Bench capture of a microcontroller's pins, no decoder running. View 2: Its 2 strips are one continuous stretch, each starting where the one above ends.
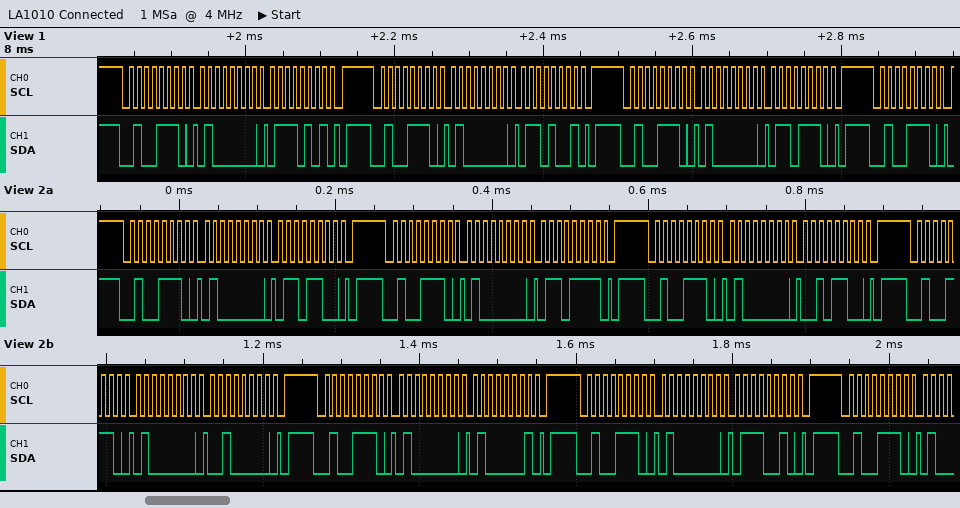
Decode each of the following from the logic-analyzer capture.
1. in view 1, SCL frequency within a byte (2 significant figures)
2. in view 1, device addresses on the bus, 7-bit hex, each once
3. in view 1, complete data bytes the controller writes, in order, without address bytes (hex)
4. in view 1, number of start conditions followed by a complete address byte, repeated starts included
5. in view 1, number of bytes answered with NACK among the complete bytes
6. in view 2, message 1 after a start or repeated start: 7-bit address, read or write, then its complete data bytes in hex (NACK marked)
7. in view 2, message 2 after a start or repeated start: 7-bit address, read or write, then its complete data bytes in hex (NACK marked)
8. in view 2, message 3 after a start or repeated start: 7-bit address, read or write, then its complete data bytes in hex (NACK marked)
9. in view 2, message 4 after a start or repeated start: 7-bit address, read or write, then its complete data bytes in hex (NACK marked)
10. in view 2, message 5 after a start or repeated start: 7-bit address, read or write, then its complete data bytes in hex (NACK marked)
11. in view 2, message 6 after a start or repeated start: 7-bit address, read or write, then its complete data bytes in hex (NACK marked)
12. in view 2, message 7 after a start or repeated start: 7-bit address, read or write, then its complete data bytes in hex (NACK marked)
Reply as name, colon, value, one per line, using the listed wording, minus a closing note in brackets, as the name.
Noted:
in view 1, SCL frequency within a byte: 100 kHz
in view 1, device addresses on the bus, 7-bit hex, each once: 0x27
in view 1, complete data bytes the controller writes, in order, without address bytes: 40 75 40 69 40 6E
in view 1, number of start conditions followed by a complete address byte, repeated starts included: 4
in view 1, number of bytes answered with NACK among the complete bytes: 0
in view 2, message 1 after a start or repeated start: 7-bit address, read or write, then its complete data bytes in hex: 0x27 write: 40 6C
in view 2, message 2 after a start or repeated start: 7-bit address, read or write, then its complete data bytes in hex: 0x27 write: 40 6F
in view 2, message 3 after a start or repeated start: 7-bit address, read or write, then its complete data bytes in hex: 0x27 write: 40 2C
in view 2, message 4 after a start or repeated start: 7-bit address, read or write, then its complete data bytes in hex: 0x27 write: 40 20
in view 2, message 5 after a start or repeated start: 7-bit address, read or write, then its complete data bytes in hex: 0x27 write: 40 41
in view 2, message 6 after a start or repeated start: 7-bit address, read or write, then its complete data bytes in hex: 0x27 write: 40 72
in view 2, message 7 after a start or repeated start: 7-bit address, read or write, then its complete data bytes in hex: 0x27 write
